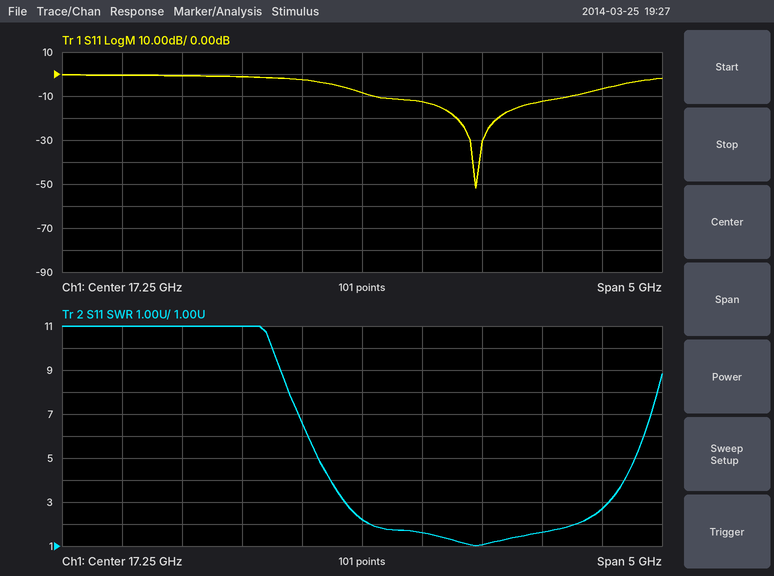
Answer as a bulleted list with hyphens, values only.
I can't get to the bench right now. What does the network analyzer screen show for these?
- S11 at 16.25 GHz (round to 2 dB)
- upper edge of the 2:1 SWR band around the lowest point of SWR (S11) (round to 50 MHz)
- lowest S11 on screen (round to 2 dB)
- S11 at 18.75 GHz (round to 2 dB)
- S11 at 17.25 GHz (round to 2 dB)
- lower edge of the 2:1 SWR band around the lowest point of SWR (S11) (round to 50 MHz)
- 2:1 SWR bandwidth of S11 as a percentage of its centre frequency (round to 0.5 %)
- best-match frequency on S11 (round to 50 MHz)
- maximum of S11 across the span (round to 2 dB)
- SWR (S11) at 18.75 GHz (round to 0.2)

- -2 dB
- 19.05 GHz
- -52 dB
- -12 dB
- -8 dB
- 17.30 GHz
- 9.5 %
- 18.20 GHz
- 0 dB
- 1.6
